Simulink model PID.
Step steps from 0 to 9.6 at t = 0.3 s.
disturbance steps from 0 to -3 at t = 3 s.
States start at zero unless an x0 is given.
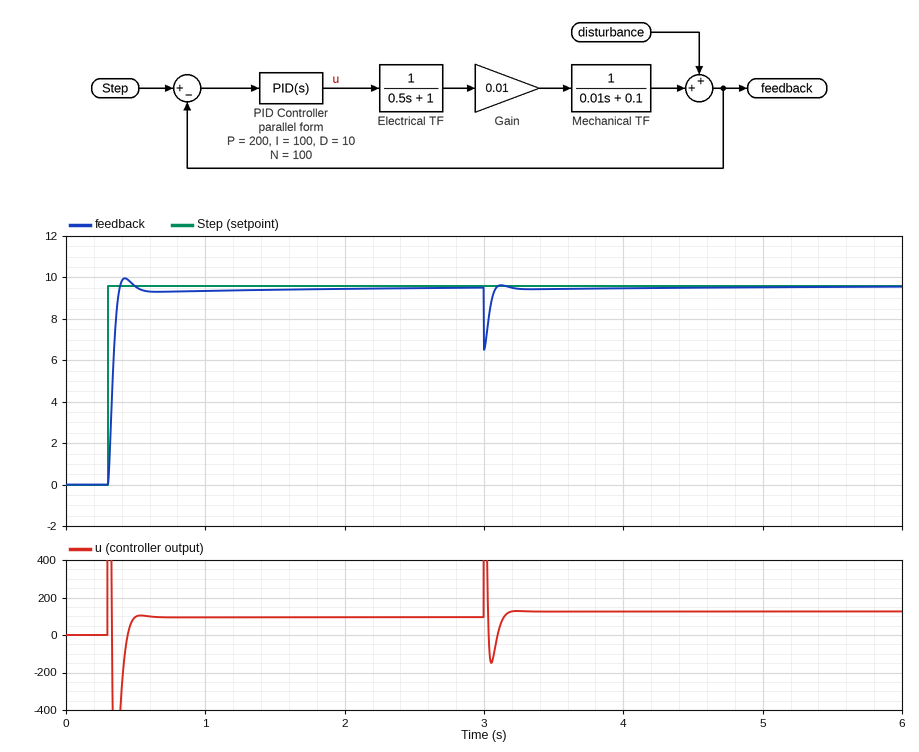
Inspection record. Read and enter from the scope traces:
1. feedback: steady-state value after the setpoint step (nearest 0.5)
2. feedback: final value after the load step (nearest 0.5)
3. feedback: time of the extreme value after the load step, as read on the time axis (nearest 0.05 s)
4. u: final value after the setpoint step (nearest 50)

9.5
9.5
3.00 s
100
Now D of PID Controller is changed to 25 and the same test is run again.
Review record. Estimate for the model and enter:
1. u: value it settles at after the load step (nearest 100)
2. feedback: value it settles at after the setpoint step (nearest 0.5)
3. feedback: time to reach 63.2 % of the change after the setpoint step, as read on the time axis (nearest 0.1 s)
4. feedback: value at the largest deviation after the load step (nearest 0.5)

100
9.5
0.3 s
6.5
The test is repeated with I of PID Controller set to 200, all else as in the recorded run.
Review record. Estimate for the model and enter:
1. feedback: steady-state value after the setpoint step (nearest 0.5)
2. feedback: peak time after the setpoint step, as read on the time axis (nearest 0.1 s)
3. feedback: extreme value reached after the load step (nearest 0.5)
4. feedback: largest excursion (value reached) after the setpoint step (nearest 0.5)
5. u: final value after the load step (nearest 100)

9.5
0.4 s
6.5
10.0
100
